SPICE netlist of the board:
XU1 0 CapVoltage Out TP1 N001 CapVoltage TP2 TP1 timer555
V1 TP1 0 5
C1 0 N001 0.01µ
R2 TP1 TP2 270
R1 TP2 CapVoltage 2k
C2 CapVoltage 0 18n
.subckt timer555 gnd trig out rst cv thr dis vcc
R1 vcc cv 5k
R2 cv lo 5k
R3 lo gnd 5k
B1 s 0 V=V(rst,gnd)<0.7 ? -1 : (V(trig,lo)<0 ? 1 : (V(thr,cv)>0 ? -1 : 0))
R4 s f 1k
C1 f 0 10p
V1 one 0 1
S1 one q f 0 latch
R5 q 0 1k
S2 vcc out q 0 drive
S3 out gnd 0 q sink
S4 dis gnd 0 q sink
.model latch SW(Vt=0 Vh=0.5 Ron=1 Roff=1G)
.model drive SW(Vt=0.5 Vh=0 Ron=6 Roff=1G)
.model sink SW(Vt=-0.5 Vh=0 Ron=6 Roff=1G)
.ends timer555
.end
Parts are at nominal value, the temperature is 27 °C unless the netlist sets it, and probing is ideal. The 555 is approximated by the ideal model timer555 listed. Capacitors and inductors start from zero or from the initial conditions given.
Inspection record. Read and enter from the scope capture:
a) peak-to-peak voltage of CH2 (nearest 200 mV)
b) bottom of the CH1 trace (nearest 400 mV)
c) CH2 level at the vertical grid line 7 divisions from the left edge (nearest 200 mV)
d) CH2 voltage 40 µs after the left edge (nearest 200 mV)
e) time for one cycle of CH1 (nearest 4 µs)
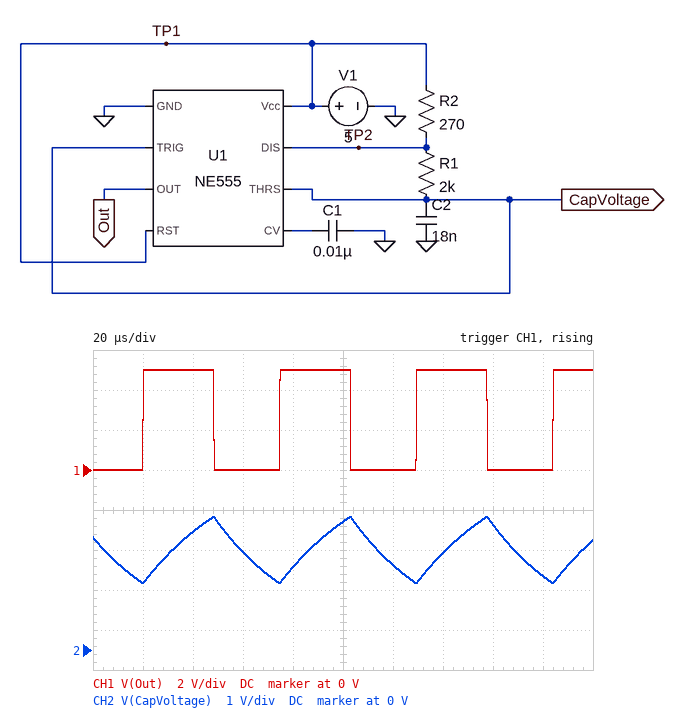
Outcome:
1.6 V
0 V
2.4 V
3.0 V
56 µs
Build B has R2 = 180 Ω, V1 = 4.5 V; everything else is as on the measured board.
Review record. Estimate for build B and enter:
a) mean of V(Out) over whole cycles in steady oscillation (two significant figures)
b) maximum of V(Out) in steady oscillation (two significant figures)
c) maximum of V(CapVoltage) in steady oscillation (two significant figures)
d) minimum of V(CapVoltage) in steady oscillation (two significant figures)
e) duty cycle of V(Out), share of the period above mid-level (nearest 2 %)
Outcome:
2.3 V
4.5 V
3.0 V
1.5 V
50 %
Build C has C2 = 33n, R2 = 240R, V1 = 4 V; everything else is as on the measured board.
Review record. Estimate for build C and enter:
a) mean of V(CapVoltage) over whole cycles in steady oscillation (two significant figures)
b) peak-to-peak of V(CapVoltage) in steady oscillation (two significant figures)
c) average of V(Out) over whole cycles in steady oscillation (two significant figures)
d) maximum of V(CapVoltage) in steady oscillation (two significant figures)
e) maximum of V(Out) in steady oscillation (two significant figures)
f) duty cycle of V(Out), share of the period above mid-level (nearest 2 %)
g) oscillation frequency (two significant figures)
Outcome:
2.0 V
1.3 V
2.1 V
2.7 V
4.0 V
52 %
10 kHz
